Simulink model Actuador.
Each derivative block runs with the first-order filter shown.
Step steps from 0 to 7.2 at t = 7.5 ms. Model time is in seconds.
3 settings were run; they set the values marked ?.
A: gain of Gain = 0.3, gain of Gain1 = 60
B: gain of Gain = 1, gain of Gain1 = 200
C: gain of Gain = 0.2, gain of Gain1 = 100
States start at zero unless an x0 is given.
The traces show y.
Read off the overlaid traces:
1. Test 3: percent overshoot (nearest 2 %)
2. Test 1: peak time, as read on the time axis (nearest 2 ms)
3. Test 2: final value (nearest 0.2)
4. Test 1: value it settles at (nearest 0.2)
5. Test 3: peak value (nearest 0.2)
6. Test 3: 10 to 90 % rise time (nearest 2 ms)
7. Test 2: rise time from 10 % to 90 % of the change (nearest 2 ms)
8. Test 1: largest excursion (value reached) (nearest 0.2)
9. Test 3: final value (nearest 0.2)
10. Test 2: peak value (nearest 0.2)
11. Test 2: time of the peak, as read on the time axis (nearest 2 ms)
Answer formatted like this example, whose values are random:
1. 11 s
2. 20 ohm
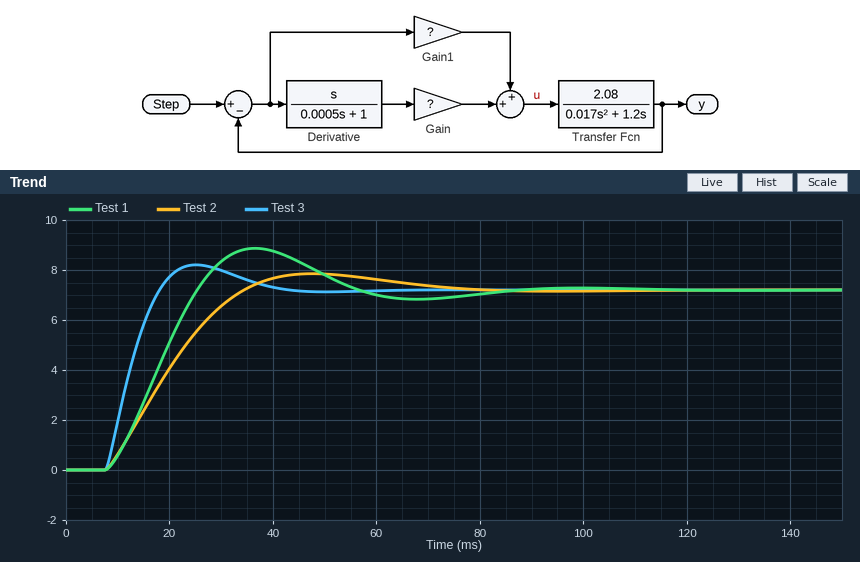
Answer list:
1. 14 %
2. 36 ms
3. 7.2
4. 7.2
5. 8.2
6. 8 ms
7. 20 ms
8. 8.8
9. 7.2
10. 7.8
11. 48 ms
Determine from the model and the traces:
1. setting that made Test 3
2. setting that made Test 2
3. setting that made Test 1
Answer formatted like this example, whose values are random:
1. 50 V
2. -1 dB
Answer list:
1. B
2. A
3. C
